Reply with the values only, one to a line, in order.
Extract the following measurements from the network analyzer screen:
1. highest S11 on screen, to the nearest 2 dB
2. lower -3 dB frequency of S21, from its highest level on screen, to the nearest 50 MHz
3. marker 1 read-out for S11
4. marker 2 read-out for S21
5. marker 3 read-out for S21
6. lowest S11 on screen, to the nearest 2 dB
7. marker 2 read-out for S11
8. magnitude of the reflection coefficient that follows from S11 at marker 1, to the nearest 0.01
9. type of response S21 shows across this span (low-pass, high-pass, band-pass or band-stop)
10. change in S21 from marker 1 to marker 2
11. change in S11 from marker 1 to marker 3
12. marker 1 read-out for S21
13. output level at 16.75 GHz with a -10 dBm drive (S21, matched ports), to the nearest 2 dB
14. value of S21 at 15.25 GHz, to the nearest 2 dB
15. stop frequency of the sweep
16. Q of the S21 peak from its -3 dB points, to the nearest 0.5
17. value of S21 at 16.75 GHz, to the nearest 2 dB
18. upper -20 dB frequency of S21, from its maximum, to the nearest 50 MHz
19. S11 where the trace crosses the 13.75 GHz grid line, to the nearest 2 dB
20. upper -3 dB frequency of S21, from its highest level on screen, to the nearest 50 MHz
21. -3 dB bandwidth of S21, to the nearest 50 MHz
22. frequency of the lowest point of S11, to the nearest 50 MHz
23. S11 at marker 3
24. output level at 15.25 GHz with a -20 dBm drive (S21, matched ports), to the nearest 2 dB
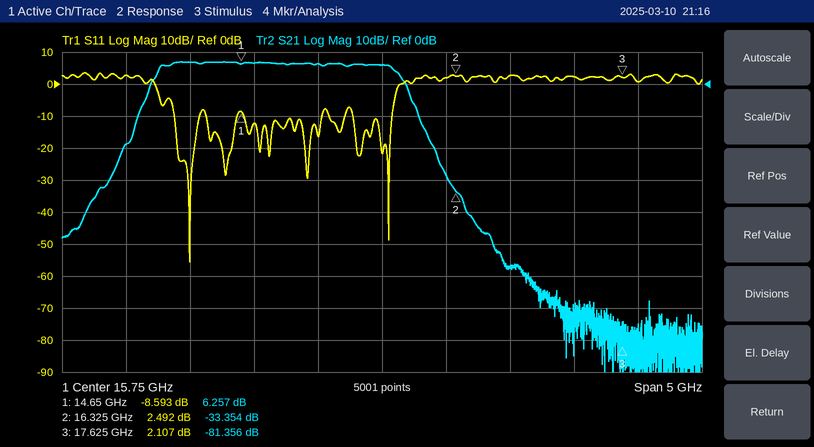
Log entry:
4 dB
14.00 GHz
-8.593 dB
-33.354 dB
-81.356 dB
-56 dB
2.492 dB
0.37
band-pass
-39.611 dB
10.700 dB
6.257 dB
-68 dBm
6 dB
18.25 GHz
8.0
-58 dB
16.05 GHz
2 dB
15.85 GHz
1.85 GHz
14.25 GHz
2.107 dB
-14 dBm
